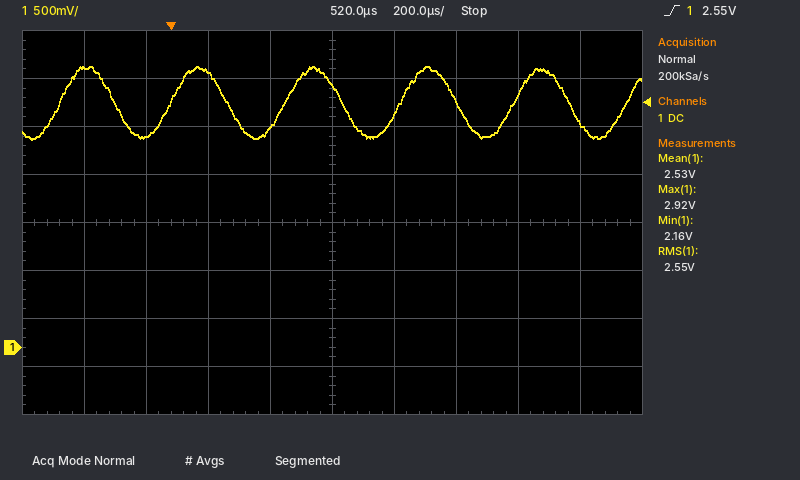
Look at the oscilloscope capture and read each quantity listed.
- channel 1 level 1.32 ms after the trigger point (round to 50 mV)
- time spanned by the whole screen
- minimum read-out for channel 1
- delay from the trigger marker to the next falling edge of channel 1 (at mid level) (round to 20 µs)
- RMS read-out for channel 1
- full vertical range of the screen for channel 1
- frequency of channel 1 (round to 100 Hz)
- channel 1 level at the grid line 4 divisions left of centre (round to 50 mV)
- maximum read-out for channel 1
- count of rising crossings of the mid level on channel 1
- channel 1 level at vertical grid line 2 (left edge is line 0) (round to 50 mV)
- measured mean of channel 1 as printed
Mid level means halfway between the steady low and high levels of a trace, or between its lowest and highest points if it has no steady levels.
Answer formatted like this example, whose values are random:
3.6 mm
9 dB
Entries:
2.35 V
2 ms
2.16 V
180 µs
2.55 V
4 V
2.7 kHz
2.90 V
2.92 V
6
2.20 V
2.53 V
